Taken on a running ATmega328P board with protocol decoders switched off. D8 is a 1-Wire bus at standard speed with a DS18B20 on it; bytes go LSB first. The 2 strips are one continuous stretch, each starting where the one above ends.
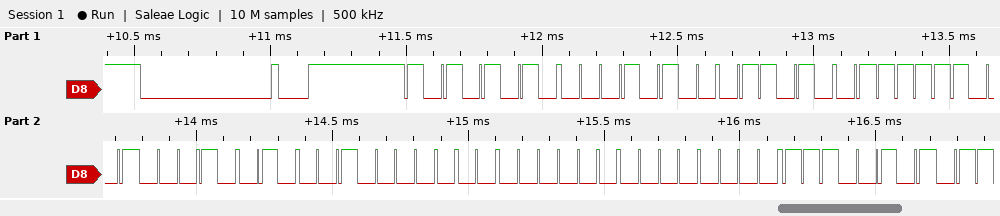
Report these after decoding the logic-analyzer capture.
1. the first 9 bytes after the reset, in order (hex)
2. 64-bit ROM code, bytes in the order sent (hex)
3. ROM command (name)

55 28 96 9F 48 04 00 00 A7
28 96 9F 48 04 00 00 A7
Match ROM
